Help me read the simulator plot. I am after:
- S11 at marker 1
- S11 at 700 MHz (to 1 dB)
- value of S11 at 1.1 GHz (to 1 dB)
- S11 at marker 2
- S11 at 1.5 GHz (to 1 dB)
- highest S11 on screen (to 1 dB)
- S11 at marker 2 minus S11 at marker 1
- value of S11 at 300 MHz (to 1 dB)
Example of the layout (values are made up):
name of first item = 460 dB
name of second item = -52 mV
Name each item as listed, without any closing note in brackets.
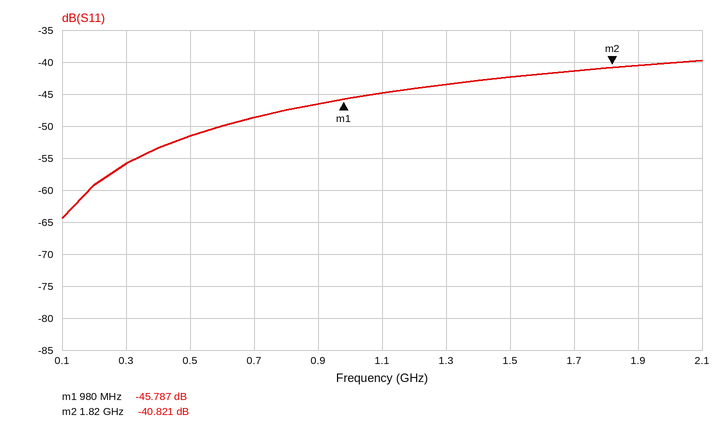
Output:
S11 at marker 1 = -45.787 dB
S11 at 700 MHz = -49 dB
value of S11 at 1.1 GHz = -45 dB
S11 at marker 2 = -40.821 dB
S11 at 1.5 GHz = -42 dB
highest S11 on screen = -40 dB
S11 at marker 2 minus S11 at marker 1 = 4.966 dB
value of S11 at 300 MHz = -56 dB
